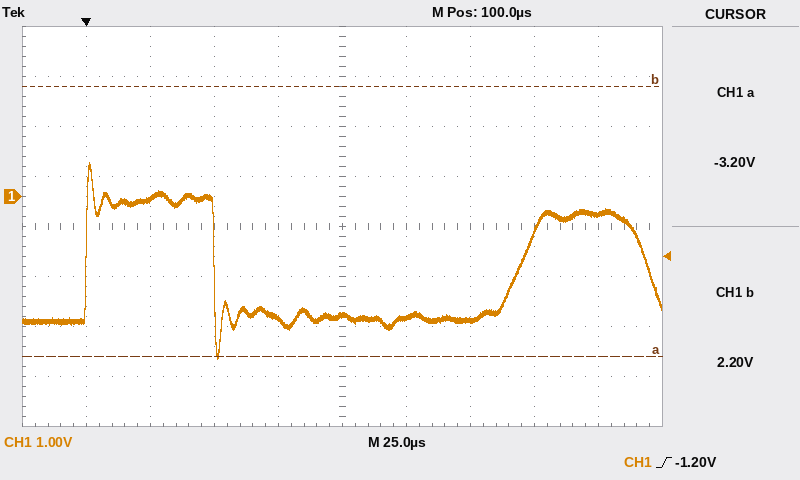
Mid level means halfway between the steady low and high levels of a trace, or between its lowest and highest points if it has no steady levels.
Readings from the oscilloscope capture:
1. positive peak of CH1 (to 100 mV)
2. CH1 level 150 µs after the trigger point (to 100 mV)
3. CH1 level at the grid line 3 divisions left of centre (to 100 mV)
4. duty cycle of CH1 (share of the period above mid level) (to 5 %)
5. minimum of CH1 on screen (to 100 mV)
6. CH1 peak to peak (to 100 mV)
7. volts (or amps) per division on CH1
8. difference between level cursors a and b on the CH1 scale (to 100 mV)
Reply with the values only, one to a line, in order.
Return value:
700 mV
-2.5 V
0.0 V
30 %
-3.2 V
3.9 V
1 V
5.4 V
